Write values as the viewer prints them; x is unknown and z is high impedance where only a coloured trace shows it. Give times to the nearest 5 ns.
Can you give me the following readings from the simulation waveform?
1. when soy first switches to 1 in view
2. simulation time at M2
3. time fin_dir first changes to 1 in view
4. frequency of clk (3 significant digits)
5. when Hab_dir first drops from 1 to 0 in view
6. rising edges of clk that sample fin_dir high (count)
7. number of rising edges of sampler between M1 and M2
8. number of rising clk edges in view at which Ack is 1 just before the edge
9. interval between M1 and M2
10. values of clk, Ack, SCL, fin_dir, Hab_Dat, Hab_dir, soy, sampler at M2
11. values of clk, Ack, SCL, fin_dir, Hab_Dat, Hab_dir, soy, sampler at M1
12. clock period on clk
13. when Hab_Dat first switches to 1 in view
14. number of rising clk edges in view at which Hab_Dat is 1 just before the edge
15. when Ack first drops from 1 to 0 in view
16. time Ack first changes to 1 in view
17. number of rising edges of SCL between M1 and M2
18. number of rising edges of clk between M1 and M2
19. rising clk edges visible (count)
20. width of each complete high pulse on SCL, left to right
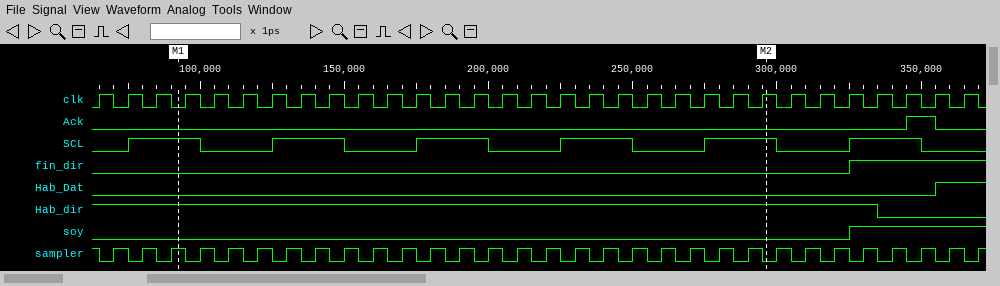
325 ns
295 ns
325 ns
100 MHz
335 ns
4
20
1
205 ns
clk=1, Ack=0, SCL=1, fin_dir=0, Hab_Dat=0, Hab_dir=1, soy=0, sampler=0
clk=0, Ack=0, SCL=1, fin_dir=0, Hab_Dat=0, Hab_dir=1, soy=0, sampler=1
10 ns
355 ns
1
355 ns
345 ns
4
21
31
25 ns, 25 ns, 25 ns, 25 ns, 25 ns, 25 ns
